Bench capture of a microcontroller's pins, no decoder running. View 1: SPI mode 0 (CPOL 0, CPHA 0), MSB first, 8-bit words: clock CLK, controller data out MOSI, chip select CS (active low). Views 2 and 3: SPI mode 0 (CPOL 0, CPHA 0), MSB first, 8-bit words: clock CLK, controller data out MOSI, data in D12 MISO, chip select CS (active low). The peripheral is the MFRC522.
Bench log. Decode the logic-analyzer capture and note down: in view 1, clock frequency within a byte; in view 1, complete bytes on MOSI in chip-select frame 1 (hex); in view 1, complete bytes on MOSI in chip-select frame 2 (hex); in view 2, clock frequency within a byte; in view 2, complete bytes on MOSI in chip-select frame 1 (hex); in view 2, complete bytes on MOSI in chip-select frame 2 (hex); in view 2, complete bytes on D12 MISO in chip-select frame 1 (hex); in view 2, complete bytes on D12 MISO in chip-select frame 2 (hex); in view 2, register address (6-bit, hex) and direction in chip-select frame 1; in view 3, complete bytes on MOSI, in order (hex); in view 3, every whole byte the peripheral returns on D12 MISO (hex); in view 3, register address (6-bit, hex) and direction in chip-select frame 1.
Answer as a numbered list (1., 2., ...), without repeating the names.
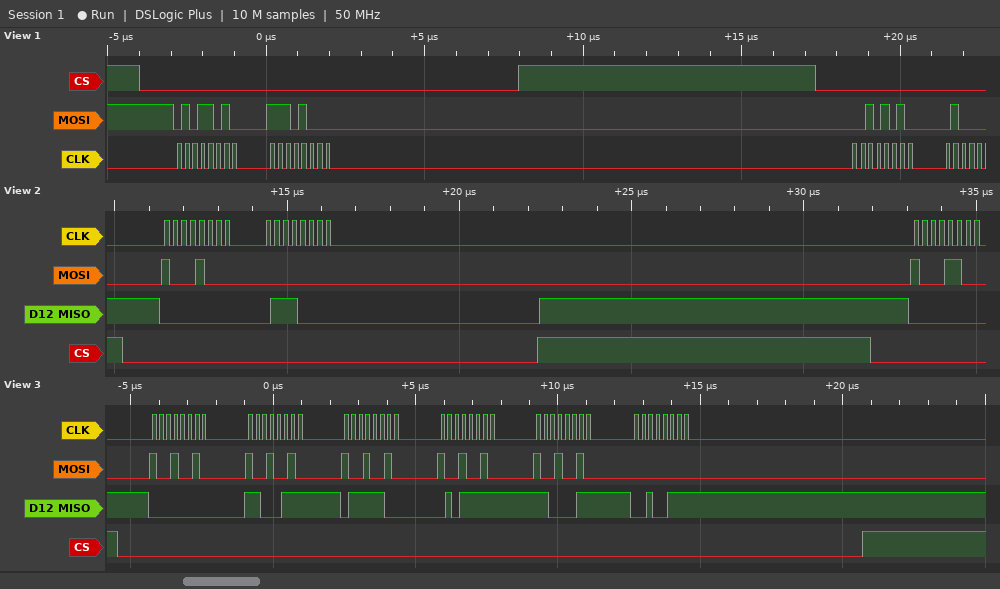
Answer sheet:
1. 4 MHz
2. 5A E8
3. 2A
4. 4 MHz
5. 88 00
6. 8C
7. 00 70
8. 00
9. 0x04 read
10. 0x92 0x92 0x92 0x92 0x92 0x00
11. 0x00 0xC7 0x7C 0x5F 0xC3 0x27
12. 0x09 read
